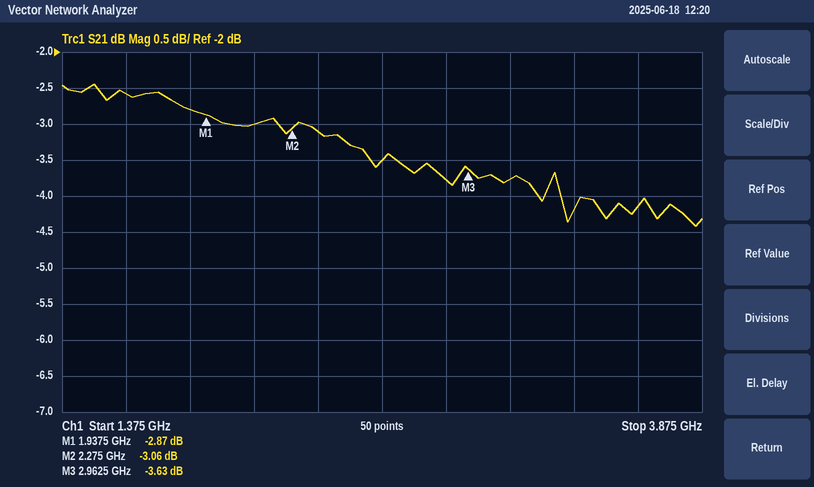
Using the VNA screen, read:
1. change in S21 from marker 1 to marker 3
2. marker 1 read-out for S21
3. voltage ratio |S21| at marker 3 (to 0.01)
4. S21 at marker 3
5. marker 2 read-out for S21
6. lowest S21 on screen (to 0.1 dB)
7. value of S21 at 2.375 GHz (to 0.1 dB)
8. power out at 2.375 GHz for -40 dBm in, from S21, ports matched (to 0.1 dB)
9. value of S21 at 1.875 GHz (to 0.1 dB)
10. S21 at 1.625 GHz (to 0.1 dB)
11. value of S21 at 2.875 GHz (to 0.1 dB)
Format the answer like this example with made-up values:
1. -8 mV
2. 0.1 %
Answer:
1. -0.76 dB
2. -2.87 dB
3. 0.66
4. -3.63 dB
5. -3.06 dB
6. -4.4 dB
7. -3.1 dB
8. -43.1 dBm
9. -2.8 dB
10. -2.6 dB
11. -3.8 dB
